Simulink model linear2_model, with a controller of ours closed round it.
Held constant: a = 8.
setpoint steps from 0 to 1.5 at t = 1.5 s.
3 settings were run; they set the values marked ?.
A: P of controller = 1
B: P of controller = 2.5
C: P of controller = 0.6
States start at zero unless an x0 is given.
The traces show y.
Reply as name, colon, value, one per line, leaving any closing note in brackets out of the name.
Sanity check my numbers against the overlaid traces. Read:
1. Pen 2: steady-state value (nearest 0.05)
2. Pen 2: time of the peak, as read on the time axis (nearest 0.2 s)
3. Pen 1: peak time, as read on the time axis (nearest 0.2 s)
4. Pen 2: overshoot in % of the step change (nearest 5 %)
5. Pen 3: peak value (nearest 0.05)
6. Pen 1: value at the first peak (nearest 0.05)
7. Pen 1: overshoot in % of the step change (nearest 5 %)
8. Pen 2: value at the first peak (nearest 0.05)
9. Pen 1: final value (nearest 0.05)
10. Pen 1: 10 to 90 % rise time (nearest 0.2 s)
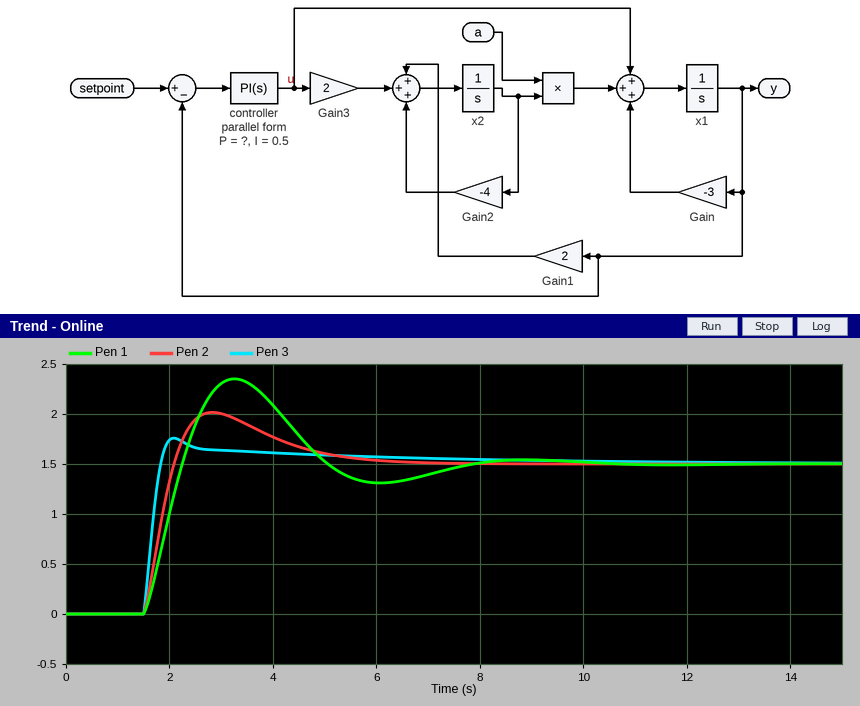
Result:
Pen 2: steady-state value: 1.50
Pen 2: time of the peak, as read on the time axis: 2.8 s
Pen 1: peak time, as read on the time axis: 3.2 s
Pen 2: overshoot in % of the step change: 35 %
Pen 3: peak value: 1.75
Pen 1: value at the first peak: 2.35
Pen 1: overshoot in % of the step change: 55 %
Pen 2: value at the first peak: 2.00
Pen 1: final value: 1.50
Pen 1: 10 to 90 % rise time: 0.6 s
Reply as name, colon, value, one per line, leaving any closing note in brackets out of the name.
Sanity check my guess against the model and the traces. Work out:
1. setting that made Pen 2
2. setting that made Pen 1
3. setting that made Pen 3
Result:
setting that made Pen 2: A
setting that made Pen 1: C
setting that made Pen 3: B
